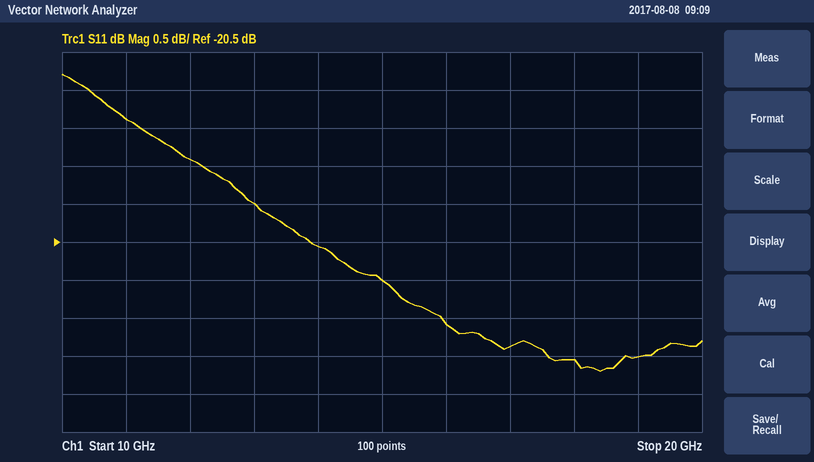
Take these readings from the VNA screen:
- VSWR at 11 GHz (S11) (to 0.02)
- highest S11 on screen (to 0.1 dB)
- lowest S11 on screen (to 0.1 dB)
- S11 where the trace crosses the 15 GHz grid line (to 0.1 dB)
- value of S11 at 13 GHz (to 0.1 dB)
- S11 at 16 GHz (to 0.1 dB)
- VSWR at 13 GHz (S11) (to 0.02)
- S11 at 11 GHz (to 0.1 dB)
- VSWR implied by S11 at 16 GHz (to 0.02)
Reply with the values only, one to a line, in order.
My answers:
1.26
-18.3 dB
-22.2 dB
-21.0 dB
-20.0 dB
-21.6 dB
1.22
-18.9 dB
1.18
